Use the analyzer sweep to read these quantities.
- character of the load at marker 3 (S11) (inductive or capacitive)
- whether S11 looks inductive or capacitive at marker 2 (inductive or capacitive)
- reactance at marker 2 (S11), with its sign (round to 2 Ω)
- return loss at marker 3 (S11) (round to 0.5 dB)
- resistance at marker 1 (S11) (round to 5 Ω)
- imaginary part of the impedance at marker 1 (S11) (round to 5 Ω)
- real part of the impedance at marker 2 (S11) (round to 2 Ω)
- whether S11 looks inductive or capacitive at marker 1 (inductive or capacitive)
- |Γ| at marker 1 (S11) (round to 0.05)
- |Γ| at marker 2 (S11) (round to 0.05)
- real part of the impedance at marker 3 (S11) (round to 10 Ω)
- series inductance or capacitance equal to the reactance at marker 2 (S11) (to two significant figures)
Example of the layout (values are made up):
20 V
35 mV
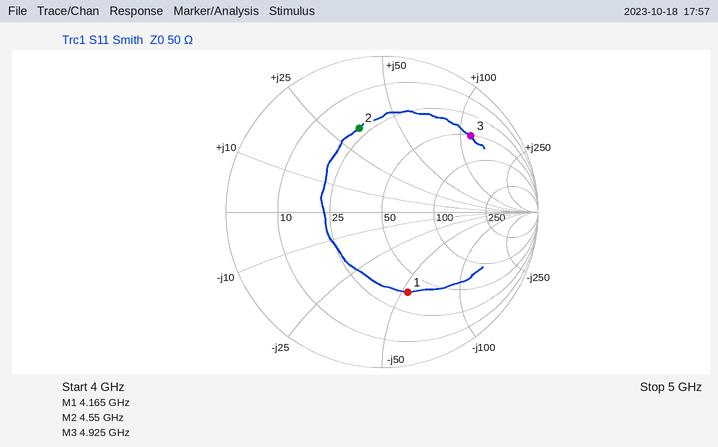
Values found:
inductive
inductive
+34 Ω
2.5 dB
35 Ω
-55 Ω
22 Ω
capacitive
0.55
0.55
50 Ω
1.2 nH
